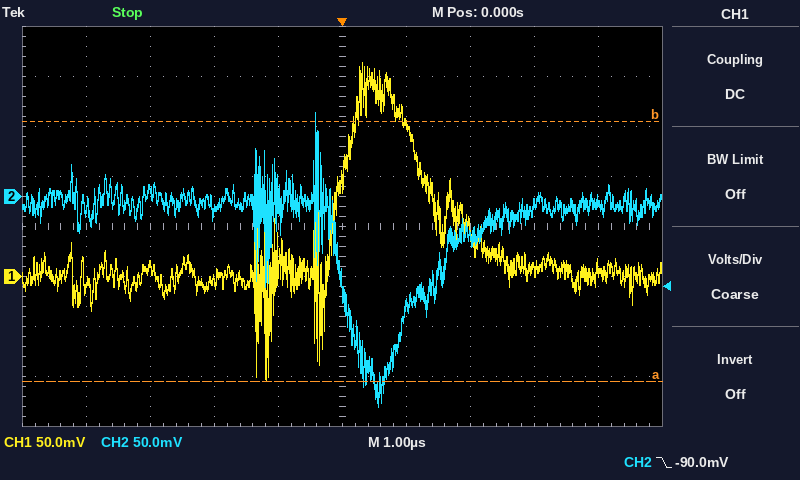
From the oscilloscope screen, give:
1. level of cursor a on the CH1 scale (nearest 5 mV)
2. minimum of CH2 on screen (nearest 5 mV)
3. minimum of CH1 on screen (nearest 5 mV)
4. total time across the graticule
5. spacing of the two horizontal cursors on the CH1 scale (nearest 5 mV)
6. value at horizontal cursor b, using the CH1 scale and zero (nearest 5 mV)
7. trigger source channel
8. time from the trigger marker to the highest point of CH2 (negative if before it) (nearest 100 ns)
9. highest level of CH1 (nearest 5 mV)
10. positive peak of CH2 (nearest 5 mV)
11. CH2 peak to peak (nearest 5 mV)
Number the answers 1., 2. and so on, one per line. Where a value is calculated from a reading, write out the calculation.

1. -105 mV
2. -210 mV
3. -105 mV
4. 10 µs
5. 260 mV
6. 155 mV
7. CH2
8. -400 ns
9. 215 mV
10. 85 mV
11. 85 mV − (-210 mV) = 295 mV
